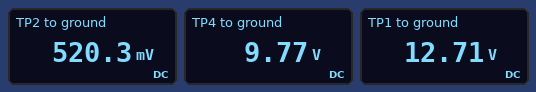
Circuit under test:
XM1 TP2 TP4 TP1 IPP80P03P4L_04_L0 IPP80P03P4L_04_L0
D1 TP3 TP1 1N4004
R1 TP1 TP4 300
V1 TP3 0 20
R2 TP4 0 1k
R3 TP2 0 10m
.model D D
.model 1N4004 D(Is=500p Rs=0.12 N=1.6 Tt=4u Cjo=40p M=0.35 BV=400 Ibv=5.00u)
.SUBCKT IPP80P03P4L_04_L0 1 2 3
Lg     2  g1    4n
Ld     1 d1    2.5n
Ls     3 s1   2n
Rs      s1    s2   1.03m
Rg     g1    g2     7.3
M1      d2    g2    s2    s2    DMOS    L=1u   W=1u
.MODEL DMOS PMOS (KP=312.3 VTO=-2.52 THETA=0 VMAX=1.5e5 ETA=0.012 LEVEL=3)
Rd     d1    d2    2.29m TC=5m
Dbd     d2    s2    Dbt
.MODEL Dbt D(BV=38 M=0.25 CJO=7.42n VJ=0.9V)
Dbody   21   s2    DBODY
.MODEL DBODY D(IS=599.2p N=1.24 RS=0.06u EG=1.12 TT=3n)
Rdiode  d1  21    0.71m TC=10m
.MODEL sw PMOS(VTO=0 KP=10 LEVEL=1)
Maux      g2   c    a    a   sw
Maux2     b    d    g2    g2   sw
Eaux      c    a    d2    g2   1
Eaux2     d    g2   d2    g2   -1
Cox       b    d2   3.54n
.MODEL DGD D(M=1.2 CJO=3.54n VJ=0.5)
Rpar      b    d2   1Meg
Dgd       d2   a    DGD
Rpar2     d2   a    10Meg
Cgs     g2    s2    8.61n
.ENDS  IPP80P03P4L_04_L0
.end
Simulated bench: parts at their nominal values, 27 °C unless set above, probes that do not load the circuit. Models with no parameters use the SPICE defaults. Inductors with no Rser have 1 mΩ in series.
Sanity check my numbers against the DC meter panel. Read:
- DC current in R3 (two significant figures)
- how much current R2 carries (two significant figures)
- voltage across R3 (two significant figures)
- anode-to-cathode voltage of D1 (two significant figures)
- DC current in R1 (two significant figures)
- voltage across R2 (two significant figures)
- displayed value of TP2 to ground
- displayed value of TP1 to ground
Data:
52 A
9.8 mA
520 mV
7.3 V
9.8 mA
9.8 V
520.3 mV
12.71 V
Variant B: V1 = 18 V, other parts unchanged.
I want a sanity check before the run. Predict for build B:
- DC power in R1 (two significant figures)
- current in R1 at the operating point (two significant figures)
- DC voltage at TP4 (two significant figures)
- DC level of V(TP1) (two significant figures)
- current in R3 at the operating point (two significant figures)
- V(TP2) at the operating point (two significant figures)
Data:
27 mW
9.4 mA
9.4 V
12 V
39 A
390 mV
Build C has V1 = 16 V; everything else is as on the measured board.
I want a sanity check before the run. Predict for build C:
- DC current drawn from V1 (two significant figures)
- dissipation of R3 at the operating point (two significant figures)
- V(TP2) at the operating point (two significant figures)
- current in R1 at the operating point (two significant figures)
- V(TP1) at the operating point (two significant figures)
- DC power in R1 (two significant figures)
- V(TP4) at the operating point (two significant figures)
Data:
27 A
7.3 W
270 mV
9.0 mA
12 V
24 mW
9.0 V
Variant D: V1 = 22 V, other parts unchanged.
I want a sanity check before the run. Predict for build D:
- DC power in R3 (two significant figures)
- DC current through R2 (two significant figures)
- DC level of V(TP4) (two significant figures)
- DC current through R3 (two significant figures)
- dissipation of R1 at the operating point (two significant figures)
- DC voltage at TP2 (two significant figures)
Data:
42 W
10 mA
10 V
65 A
31 mW
650 mV
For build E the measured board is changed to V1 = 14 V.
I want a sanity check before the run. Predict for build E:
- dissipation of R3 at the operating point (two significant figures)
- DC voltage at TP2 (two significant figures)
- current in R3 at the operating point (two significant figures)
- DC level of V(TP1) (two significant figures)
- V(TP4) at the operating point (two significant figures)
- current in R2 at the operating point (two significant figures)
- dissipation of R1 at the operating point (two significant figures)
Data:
2.4 W
150 mV
15 A
11 V
8.6 V
8.6 mA
22 mW
